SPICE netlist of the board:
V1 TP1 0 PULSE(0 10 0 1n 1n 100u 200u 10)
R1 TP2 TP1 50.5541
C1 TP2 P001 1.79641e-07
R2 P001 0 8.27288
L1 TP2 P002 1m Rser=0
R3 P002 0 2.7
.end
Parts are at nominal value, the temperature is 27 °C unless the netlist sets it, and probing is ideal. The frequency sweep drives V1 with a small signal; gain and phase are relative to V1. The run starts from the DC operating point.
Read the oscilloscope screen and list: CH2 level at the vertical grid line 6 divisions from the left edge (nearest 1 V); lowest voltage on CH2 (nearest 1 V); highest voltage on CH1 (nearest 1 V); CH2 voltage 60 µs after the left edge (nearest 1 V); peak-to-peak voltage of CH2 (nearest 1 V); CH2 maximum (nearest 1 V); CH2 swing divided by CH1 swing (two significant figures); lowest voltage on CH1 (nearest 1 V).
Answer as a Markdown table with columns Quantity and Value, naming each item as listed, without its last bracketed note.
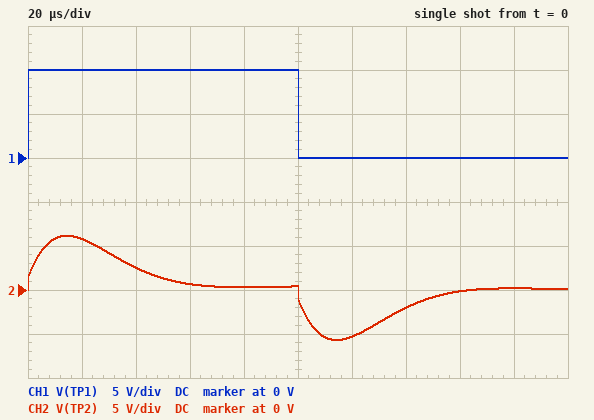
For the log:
| Quantity | Value |
|---|---|
| CH2 level at the vertical grid line 6 divisions from the left edge | -5 V |
| lowest voltage on CH2 | -6 V |
| highest voltage on CH1 | 10 V |
| CH2 voltage 60 µs after the left edge | 1 V |
| peak-to-peak voltage of CH2 | 12 V |
| CH2 maximum | 6 V |
| CH2 swing divided by CH1 swing | 1.2 |
| lowest voltage on CH1 | 0 V |
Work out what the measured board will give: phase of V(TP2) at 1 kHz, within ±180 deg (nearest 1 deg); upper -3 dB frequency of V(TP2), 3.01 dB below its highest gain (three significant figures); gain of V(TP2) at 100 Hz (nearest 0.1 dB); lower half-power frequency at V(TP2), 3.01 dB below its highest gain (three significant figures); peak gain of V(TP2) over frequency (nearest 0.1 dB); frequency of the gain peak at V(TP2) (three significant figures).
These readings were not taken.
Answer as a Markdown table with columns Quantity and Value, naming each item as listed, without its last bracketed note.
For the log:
| Quantity | Value |
|---|---|
| phase of V(TP2) at 1 kHz, within ±180 deg | 60 deg |
| upper -3 dB frequency of V(TP2), 3.01 dB below its highest gain | 22.8 kHz |
| gain of V(TP2) at 100 Hz | -25.7 dB |
| lower half-power frequency at V(TP2), 3.01 dB below its highest gain | 5.73 kHz |
| peak gain of V(TP2) over frequency | -0.8 dB |
| frequency of the gain peak at V(TP2) | 11.4 kHz |
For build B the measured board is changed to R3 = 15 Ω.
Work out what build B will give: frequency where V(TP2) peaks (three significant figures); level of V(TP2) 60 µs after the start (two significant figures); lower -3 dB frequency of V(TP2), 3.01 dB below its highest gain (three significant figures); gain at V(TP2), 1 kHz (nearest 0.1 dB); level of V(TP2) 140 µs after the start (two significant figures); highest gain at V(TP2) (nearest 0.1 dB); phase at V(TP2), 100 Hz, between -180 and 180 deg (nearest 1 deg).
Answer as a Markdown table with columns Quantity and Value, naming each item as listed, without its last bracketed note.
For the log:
| Quantity | Value |
|---|---|
| frequency where V(TP2) peaks | 12.4 kHz |
| level of V(TP2) 60 µs after the start | 2.3 V |
| lower -3 dB frequency of V(TP2), 3.01 dB below its highest gain | 5.94 kHz |
| gain at V(TP2), 1 kHz | -12.1 dB |
| level of V(TP2) 140 µs after the start | -1.2 V |
| highest gain at V(TP2) | -1.6 dB |
| phase at V(TP2), 100 Hz, between -180 and 180 deg | 2 deg |
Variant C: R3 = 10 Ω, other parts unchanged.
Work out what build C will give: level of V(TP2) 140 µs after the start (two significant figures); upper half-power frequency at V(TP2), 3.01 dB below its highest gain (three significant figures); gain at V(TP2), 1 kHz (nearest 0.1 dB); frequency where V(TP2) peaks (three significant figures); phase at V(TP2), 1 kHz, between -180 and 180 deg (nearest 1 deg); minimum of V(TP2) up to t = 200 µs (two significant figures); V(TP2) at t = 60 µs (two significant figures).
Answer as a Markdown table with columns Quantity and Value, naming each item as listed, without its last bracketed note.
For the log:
| Quantity | Value |
|---|---|
| level of V(TP2) 140 µs after the start | -1.5 V |
| upper half-power frequency at V(TP2), 3.01 dB below its highest gain | 24.2 kHz |
| gain at V(TP2), 1 kHz | -14.2 dB |
| frequency where V(TP2) peaks | 12.0 kHz |
| phase at V(TP2), 1 kHz, between -180 and 180 deg | 26 deg |
| minimum of V(TP2) up to t = 200 µs | -4.6 V |
| V(TP2) at t = 60 µs | 1.7 V |
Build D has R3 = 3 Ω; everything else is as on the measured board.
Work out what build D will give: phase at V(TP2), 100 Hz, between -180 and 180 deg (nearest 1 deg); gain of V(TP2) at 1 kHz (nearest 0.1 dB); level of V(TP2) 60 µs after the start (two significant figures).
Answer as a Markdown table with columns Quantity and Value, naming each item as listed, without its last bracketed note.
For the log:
| Quantity | Value |
|---|---|
| phase at V(TP2), 100 Hz, between -180 and 180 deg | 11 deg |
| gain of V(TP2) at 1 kHz | -17.7 dB |
| level of V(TP2) 60 µs after the start | 710 mV |
